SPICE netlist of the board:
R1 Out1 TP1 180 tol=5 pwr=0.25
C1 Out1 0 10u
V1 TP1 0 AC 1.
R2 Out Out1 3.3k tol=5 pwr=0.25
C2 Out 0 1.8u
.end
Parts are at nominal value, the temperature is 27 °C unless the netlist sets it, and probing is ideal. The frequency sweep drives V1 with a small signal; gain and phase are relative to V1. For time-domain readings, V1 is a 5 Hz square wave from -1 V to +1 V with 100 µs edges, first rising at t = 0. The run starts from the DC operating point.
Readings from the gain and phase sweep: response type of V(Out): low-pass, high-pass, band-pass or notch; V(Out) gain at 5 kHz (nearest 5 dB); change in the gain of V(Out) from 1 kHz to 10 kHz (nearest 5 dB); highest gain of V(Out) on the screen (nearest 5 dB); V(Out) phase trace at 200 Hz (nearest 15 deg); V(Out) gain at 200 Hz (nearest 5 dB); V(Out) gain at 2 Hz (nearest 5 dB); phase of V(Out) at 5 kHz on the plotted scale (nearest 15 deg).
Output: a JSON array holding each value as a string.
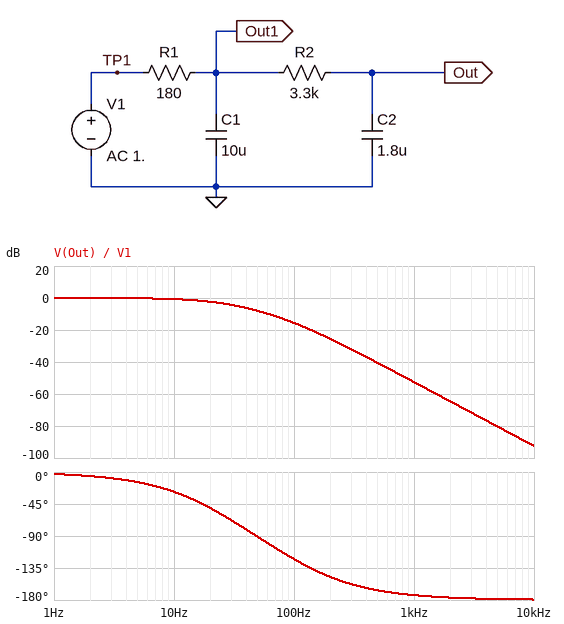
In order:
["low-pass", "-80 dB", "-40 dB", "0 dB", "-150 deg", "-25 dB", "0 dB", "-180 deg"]
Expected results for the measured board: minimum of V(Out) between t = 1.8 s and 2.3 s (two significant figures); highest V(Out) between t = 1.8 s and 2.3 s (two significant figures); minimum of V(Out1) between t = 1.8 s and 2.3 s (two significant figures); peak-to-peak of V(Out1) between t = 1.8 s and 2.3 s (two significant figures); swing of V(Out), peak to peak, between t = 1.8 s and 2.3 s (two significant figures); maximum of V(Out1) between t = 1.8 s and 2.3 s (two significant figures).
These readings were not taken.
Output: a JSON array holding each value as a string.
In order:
["-1.0 V", "1.0 V", "-1.0 V", "2.0 V", "2.0 V", "1.0 V"]
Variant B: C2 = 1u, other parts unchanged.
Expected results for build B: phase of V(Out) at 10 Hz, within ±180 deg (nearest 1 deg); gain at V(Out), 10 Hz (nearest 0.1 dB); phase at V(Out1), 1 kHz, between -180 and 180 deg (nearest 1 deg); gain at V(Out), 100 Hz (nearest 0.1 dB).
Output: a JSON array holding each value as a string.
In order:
["-19 deg", "-0.3 dB", "-85 deg", "-11.1 dB"]
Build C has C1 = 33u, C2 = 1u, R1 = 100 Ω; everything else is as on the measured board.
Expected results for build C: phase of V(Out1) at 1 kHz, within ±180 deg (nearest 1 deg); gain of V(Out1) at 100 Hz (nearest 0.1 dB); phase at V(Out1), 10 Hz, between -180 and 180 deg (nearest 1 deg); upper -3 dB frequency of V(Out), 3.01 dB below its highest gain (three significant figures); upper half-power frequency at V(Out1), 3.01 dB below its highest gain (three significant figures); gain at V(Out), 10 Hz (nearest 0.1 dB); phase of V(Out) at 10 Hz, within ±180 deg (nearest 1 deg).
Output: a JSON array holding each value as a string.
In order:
["-87 deg", "-7.3 dB", "-12 deg", "30.4 Hz", "46.8 Hz", "-0.4 dB", "-24 deg"]
